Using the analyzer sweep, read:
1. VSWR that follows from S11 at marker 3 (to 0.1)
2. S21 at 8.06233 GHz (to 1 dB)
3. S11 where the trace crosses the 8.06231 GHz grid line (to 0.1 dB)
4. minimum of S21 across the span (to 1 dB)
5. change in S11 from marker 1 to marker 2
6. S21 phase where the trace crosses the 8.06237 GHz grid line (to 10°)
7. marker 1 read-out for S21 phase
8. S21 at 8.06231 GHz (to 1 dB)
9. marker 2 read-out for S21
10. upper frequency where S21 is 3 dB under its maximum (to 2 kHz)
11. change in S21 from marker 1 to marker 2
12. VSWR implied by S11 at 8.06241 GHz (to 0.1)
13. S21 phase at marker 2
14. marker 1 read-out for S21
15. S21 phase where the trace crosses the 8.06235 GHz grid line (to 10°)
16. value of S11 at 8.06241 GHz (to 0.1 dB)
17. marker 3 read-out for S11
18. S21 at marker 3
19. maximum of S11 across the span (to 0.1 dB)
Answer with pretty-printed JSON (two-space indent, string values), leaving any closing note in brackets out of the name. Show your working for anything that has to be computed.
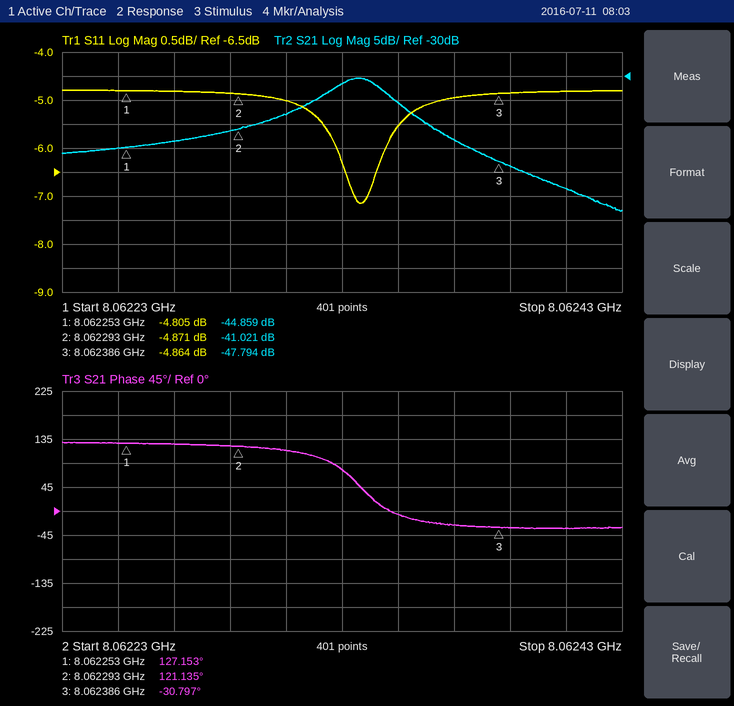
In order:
{
  "VSWR that follows from S11 at marker 3": "(1 + 0.5712)/(1 − 0.5712) ≈ 3.7",
  "S21 at 8.06233 GHz": "-32 dB",
  "S11 where the trace crosses the 8.06231 GHz grid line": "-5.0 dB",
  "minimum of S21 across the span": "-58 dB",
  "change in S11 from marker 1 to marker 2": "-4.871 − (-4.805) = -0.066 dB",
  "S21 phase where the trace crosses the 8.06237 GHz grid line": "-30°",
  "marker 1 read-out for S21 phase": "127.153°",
  "S21 at 8.06231 GHz": "-38 dB",
  "marker 2 read-out for S21": "-41.021 dB",
  "upper frequency where S21 is 3 dB under its maximum": "8.062346 GHz",
  "change in S21 from marker 1 to marker 2": "-41.021 − (-44.859) = 3.838 dB",
  "VSWR implied by S11 at 8.06241 GHz": "|Γ| = 10^(-4.8/20) = 0.5754; VSWR = (1 + 0.5754)/(1 − 0.5754) ≈ 3.7",
  "S21 phase at marker 2": "121.135°",
  "marker 1 read-out for S21": "-44.859 dB",
  "S21 phase where the trace crosses the 8.06235 GHz grid line": "-10°",
  "value of S11 at 8.06241 GHz": "-4.8 dB",
  "marker 3 read-out for S11": "-4.864 dB",
  "S21 at marker 3": "-47.794 dB",
  "maximum of S11 across the span": "-4.8 dB"
}
